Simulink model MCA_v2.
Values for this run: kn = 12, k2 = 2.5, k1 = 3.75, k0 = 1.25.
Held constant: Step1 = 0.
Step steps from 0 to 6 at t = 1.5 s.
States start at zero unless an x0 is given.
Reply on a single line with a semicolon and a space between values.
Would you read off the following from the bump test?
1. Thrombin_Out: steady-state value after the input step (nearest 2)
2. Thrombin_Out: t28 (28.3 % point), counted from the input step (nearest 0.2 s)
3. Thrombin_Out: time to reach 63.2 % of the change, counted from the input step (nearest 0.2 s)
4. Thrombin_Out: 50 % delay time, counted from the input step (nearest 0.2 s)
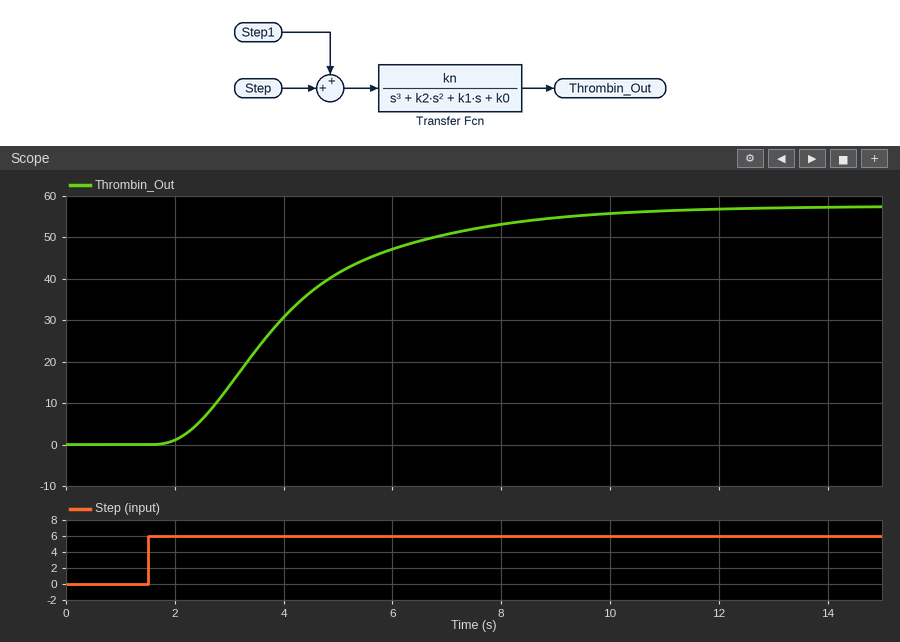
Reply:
58; 1.6 s; 3.0 s; 2.4 s
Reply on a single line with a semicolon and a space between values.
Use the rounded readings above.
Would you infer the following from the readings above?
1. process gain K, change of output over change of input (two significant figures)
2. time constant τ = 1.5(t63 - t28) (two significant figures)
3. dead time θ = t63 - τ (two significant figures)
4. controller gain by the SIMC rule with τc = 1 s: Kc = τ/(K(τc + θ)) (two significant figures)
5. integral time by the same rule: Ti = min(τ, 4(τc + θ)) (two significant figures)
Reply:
9.7; 2.1 s; 0.90 s; 0.11; 2.1 s
